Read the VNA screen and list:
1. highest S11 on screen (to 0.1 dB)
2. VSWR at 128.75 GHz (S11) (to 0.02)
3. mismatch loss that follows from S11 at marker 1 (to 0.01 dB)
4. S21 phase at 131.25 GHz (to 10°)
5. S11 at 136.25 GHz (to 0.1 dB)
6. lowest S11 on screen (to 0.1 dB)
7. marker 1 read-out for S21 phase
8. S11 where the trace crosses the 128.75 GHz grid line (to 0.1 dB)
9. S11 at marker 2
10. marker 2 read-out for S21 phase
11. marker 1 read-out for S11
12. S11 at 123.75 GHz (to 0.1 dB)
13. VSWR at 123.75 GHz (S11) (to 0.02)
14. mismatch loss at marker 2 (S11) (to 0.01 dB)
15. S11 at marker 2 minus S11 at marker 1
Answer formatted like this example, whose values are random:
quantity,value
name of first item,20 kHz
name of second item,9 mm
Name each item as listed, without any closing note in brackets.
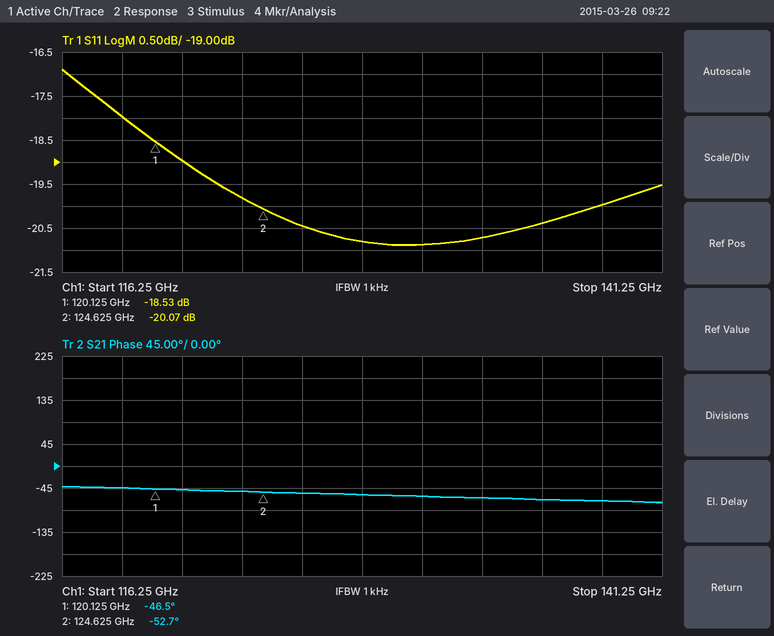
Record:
quantity,value
highest S11 on screen,-16.9 dB
VSWR at 128.75 GHz (S11),1.20
mismatch loss that follows from S11 at marker 1,0.06 dB
S21 phase at 131.25 GHz,-60°
S11 at 136.25 GHz,-20.4 dB
lowest S11 on screen,-20.9 dB
marker 1 read-out for S21 phase,-46.5°
S11 where the trace crosses the 128.75 GHz grid line,-20.8 dB
S11 at marker 2,-20.07 dB
marker 2 read-out for S21 phase,-52.7°
marker 1 read-out for S11,-18.53 dB
S11 at 123.75 GHz,-19.8 dB
VSWR at 123.75 GHz (S11),1.22
mismatch loss at marker 2 (S11),0.04 dB
S11 at marker 2 minus S11 at marker 1,-1.54 dB
